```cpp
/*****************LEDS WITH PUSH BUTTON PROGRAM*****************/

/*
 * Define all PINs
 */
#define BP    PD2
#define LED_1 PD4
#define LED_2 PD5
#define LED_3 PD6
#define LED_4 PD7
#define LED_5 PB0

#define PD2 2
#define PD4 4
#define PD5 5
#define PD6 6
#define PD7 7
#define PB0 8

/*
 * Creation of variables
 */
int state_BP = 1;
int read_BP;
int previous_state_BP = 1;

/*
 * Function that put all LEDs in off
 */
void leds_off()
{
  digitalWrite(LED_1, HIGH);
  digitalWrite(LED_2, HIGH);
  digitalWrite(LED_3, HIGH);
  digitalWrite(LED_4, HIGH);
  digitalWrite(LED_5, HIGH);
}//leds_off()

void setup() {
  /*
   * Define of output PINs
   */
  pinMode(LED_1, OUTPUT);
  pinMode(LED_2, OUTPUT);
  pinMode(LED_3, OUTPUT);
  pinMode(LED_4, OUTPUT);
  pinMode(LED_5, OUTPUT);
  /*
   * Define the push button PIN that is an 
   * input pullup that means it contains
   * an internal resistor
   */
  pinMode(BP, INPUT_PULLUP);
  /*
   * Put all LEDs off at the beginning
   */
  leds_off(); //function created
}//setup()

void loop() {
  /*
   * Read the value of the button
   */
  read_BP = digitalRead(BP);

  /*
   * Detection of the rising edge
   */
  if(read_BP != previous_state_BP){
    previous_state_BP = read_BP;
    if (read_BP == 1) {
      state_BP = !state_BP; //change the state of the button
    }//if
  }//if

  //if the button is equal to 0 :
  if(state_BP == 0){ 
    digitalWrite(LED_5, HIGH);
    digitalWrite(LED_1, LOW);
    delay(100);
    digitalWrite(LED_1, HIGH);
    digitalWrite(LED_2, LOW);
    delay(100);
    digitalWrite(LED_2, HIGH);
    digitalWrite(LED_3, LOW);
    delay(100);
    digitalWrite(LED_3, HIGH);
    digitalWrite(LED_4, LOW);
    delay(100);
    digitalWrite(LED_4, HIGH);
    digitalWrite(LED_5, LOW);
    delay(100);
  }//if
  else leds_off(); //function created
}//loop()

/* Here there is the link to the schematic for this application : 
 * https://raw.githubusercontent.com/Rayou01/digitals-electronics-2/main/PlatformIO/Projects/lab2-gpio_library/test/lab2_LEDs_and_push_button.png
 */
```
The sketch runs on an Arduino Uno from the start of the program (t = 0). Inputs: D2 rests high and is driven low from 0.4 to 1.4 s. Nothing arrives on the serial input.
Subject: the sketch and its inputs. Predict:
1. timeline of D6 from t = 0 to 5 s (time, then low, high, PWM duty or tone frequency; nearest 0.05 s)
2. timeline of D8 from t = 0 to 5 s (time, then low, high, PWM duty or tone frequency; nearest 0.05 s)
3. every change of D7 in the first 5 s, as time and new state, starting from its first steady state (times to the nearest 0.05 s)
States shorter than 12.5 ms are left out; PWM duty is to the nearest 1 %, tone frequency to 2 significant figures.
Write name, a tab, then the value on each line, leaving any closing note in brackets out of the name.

timeline of D6 from t = 0 to 5 s	0 s high; 1.6 s low; 1.7 s high; 2.1 s low; 2.2 s high; 2.6 s low; 2.7 s high; 3.1 s low; 3.2 s high; 3.6 s low; 3.7 s high; 4.1 s low; 4.2 s high; 4.6 s low; 4.7 s high
timeline of D8 from t = 0 to 5 s	0 s high; 1.8 s low; 1.9 s high; 2.3 s low; 2.4 s high; 2.8 s low; 2.9 s high; 3.3 s low; 3.4 s high; 3.8 s low; 3.9 s high; 4.3 s low; 4.4 s high; 4.8 s low; 4.9 s high
every change of D7 in the first 5 s, as time and new state, starting from its first steady state	0 s high; 1.7 s low; 1.8 s high; 2.2 s low; 2.3 s high; 2.7 s low; 2.8 s high; 3.2 s low; 3.3 s high; 3.7 s low; 3.8 s high; 4.2 s low; 4.3 s high; 4.7 s low; 4.8 s high
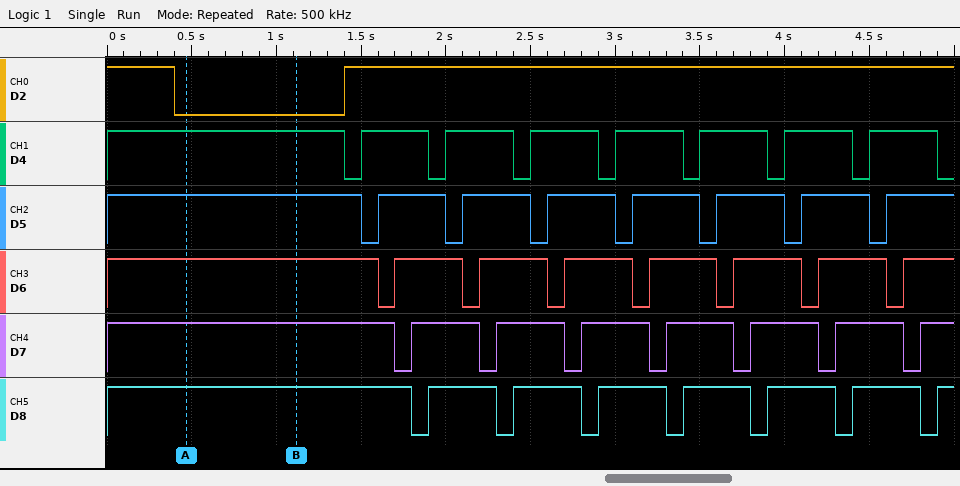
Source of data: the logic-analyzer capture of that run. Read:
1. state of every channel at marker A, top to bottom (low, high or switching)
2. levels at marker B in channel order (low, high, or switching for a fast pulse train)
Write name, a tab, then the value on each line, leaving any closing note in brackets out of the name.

state of every channel at marker A, top to bottom	D2 low, D4 high, D5 high, D6 high, D7 high, D8 high
levels at marker B in channel order	D2 low, D4 high, D5 high, D6 high, D7 high, D8 high
